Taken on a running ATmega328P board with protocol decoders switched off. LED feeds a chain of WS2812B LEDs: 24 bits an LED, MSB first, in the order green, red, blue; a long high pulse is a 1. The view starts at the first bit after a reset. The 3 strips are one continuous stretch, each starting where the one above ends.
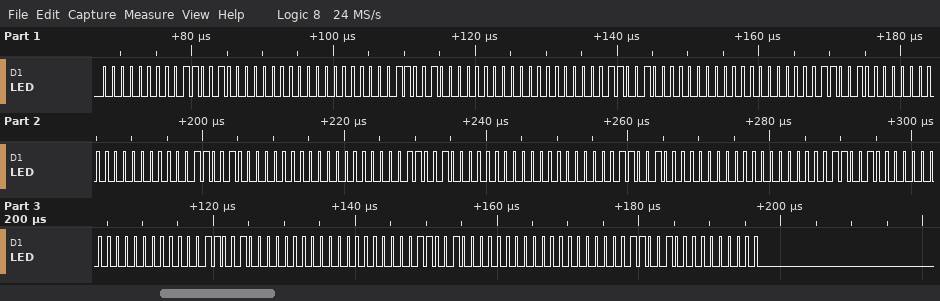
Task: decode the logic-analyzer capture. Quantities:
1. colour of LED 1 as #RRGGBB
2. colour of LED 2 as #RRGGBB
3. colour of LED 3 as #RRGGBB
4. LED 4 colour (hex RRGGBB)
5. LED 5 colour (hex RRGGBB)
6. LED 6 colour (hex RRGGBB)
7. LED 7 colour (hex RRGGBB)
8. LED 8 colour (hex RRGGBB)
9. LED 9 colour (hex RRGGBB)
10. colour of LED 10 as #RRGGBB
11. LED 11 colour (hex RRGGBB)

#640000
#640000
#640000
#640000
#640000
#640000
#640000
#640000
#640000
#640000
#640000
